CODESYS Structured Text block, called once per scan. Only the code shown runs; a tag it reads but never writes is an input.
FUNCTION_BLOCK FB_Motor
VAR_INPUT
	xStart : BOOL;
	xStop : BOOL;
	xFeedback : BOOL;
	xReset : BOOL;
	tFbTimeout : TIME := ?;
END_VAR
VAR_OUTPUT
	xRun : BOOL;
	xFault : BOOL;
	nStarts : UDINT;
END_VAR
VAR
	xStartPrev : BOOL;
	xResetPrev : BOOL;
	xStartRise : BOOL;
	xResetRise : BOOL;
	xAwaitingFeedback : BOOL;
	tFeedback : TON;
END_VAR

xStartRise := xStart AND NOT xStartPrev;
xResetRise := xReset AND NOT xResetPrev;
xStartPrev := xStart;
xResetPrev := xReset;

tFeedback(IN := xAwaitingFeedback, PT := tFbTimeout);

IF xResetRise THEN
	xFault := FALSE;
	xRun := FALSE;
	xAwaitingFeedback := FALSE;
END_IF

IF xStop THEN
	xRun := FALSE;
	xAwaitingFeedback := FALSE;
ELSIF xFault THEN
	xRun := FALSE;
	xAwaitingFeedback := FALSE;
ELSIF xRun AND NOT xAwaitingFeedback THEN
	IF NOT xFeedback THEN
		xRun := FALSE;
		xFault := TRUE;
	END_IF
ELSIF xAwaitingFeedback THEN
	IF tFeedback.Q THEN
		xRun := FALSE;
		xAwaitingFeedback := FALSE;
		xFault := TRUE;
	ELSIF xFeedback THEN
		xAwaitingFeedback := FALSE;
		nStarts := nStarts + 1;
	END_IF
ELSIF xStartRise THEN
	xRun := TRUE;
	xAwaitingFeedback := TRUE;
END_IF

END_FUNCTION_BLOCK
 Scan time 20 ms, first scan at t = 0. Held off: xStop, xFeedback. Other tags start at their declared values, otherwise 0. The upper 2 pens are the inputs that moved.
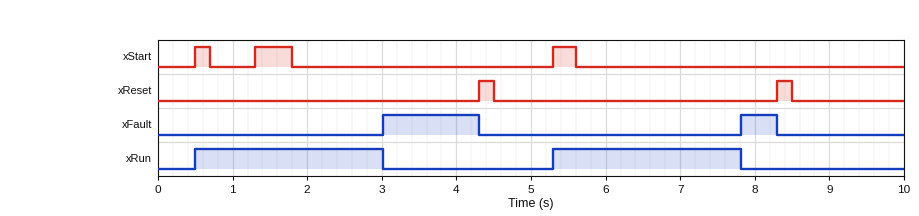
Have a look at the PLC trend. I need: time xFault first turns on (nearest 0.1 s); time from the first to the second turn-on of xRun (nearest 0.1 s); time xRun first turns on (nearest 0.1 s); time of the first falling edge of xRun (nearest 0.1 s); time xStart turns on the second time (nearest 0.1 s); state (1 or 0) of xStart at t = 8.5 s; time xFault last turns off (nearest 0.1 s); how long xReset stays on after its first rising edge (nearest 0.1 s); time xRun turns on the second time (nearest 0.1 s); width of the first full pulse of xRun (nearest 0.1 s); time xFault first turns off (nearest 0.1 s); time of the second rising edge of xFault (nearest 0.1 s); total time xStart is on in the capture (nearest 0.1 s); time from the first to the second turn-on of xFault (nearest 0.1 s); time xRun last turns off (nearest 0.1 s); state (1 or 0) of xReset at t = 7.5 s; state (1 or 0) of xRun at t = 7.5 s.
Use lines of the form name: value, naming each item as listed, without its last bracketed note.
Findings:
time xFault first turns on: 3.0 s
time from the first to the second turn-on of xRun: 4.8 s
time xRun first turns on: 0.5 s
time of the first falling edge of xRun: 3.0 s
time xStart turns on the second time: 1.3 s
state (1 or 0) of xStart at t = 8.5 s: 0
time xFault last turns off: 8.3 s
how long xReset stays on after its first rising edge: 0.2 s
time xRun turns on the second time: 5.3 s
width of the first full pulse of xRun: 2.5 s
time xFault first turns off: 4.3 s
time of the second rising edge of xFault: 7.8 s
total time xStart is on in the capture: 1.0 s
time from the first to the second turn-on of xFault: 4.8 s
time xRun last turns off: 7.8 s
state (1 or 0) of xReset at t = 7.5 s: 0
state (1 or 0) of xRun at t = 7.5 s: 1
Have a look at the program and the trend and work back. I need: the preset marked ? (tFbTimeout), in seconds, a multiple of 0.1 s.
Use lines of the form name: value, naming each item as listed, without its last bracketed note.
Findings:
the preset marked ? (tFbTimeout), in seconds, a multiple of 0.1 s: 2.5 s
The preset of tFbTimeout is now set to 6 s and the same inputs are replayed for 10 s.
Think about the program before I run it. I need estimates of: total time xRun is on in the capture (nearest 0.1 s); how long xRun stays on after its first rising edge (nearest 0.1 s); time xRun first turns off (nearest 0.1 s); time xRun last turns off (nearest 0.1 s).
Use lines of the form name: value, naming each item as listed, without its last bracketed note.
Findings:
total time xRun is on in the capture: 6.8 s
how long xRun stays on after its first rising edge: 3.8 s
time xRun first turns off: 4.3 s
time xRun last turns off: 8.3 s
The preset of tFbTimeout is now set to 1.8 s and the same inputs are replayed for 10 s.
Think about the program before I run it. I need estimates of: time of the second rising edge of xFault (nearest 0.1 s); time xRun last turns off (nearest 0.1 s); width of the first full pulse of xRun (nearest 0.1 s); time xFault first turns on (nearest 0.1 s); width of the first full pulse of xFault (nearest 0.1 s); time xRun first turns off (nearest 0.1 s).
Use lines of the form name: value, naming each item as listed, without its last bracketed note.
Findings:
time of the second rising edge of xFault: 7.1 s
time xRun last turns off: 7.1 s
width of the first full pulse of xRun: 1.8 s
time xFault first turns on: 2.3 s
width of the first full pulse of xFault: 2.0 s
time xRun first turns off: 2.3 s
